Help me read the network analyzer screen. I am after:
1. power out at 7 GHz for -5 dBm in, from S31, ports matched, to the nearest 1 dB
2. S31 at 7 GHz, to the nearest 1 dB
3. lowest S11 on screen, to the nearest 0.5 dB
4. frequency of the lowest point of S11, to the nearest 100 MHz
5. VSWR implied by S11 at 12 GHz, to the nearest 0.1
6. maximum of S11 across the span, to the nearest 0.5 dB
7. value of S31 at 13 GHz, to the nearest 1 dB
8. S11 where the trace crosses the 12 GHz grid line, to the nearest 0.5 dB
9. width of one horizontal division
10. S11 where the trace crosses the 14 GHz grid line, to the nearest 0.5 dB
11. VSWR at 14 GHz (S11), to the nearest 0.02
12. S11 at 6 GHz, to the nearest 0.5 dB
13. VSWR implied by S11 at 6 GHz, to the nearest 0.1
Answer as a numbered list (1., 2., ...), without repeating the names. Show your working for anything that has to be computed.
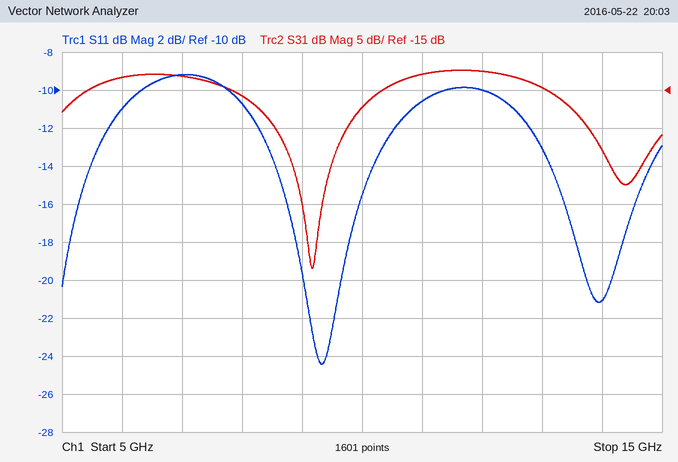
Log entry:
1. -5 dBm + (-13 dB) = -18 dBm
2. -13 dB
3. -24.5 dB
4. 9.3 GHz
5. |Γ| = 10^(-10/20) = 0.3162; VSWR = (1 + 0.3162)/(1 − 0.3162) ≈ 1.9
6. -9.0 dB
7. -15 dB
8. -10.0 dB
9. 1 GHz
10. -21.0 dB
11. |Γ| = 10^(-21/20) = 0.0891; VSWR = (1 + 0.0891)/(1 − 0.0891) ≈ 1.20
12. -11.0 dB
13. |Γ| = 10^(-11/20) = 0.2818; VSWR = (1 + 0.2818)/(1 − 0.2818) ≈ 1.8
